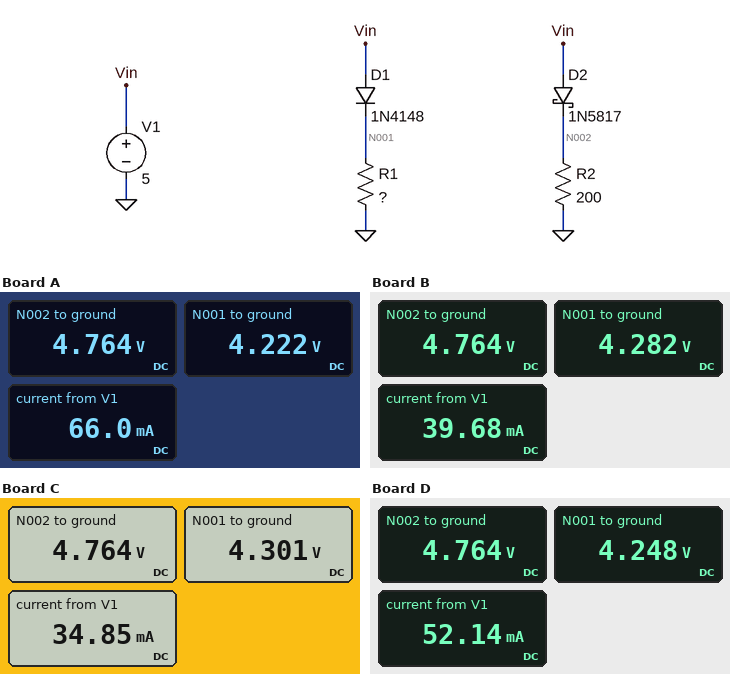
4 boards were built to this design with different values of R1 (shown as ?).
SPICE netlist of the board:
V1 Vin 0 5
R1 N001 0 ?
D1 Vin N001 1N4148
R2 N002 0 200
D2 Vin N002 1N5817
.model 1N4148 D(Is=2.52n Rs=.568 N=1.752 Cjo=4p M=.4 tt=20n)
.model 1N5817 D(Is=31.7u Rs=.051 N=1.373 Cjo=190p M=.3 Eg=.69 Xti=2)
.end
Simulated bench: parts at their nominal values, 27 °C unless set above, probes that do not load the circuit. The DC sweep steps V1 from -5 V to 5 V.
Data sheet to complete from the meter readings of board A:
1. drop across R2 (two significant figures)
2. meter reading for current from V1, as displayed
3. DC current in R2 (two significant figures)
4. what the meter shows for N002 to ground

4.8 V
66.0 mA
24 mA
4.764 V
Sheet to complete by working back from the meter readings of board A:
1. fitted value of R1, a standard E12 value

100 Ω
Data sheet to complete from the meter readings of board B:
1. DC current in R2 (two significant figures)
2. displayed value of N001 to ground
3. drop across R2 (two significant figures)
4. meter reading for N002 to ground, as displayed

24 mA
4.282 V
4.8 V
4.764 V
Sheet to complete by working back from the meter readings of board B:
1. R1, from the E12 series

270 Ω
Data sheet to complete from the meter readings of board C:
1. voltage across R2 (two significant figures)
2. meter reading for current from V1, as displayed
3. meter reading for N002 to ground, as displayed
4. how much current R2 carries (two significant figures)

4.8 V
34.85 mA
4.764 V
24 mA
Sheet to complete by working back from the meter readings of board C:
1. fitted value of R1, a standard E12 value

390 Ω
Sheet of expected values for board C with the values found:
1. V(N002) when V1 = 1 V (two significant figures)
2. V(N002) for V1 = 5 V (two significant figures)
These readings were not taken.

830 mV
4.8 V
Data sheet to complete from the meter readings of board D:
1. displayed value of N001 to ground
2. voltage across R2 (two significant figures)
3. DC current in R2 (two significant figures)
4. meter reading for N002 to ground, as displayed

4.248 V
4.8 V
24 mA
4.764 V
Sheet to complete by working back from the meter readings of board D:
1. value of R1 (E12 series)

150 Ω
